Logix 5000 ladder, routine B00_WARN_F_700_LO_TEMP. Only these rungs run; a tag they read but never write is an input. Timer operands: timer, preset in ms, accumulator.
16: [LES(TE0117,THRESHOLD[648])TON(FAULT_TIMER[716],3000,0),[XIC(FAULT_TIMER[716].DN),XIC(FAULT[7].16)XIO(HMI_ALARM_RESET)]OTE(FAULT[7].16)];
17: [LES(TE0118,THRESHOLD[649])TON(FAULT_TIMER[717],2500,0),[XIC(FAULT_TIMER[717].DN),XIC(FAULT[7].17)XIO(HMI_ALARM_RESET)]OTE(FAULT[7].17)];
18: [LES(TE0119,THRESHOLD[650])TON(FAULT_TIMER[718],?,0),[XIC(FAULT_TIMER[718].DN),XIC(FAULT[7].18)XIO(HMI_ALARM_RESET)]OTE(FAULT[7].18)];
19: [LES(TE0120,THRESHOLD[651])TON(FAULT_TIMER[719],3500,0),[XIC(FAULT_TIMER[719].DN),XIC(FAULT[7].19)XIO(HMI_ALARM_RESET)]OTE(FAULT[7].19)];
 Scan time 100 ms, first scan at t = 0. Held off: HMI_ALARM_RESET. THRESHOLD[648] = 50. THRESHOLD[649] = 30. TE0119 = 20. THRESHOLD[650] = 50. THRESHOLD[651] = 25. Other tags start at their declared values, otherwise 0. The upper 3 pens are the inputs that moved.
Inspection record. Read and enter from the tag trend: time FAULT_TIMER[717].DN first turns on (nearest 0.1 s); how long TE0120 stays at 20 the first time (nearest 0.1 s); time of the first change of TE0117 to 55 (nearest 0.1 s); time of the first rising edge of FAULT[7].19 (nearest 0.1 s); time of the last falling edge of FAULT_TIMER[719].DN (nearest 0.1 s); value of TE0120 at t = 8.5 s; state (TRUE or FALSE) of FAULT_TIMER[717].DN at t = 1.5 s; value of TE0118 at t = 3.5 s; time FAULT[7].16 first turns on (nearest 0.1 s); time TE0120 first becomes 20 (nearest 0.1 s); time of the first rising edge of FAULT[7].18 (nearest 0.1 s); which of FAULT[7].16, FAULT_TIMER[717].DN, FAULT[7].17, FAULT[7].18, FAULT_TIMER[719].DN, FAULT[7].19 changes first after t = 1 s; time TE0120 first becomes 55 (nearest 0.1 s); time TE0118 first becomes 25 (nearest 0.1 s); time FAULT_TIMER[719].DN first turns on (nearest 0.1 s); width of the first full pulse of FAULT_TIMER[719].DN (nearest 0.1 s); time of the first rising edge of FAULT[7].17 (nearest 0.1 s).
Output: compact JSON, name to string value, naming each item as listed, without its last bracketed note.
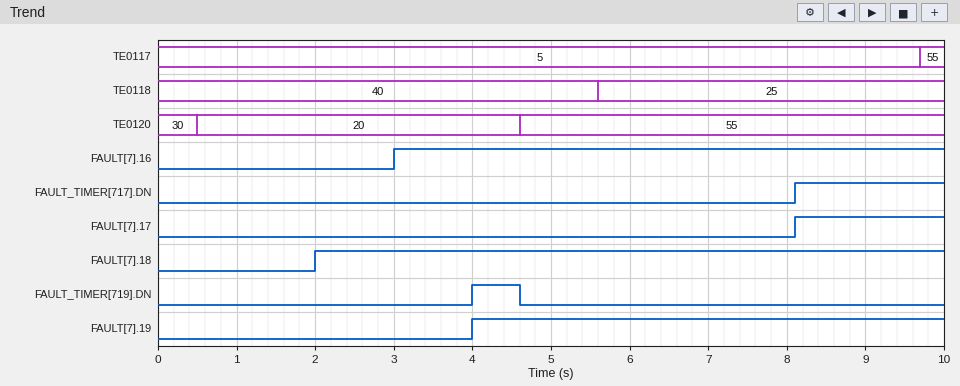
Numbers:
{"time FAULT_TIMER[717].DN first turns on": "8.1 s", "how long TE0120 stays at 20 the first time": "4.1 s", "time of the first change of TE0117 to 55": "9.7 s", "time of the first rising edge of FAULT[7].19": "4.0 s", "time of the last falling edge of FAULT_TIMER[719].DN": "4.6 s", "value of TE0120 at t = 8.5 s": "55", "state (TRUE or FALSE) of FAULT_TIMER[717].DN at t = 1.5 s": "FALSE", "value of TE0118 at t = 3.5 s": "40", "time FAULT[7].16 first turns on": "3.0 s", "time TE0120 first becomes 20": "0.5 s", "time of the first rising edge of FAULT[7].18": "2.0 s", "which of FAULT[7].16, FAULT_TIMER[717].DN, FAULT[7].17, FAULT[7].18, FAULT_TIMER[719].DN, FAULT[7].19 changes first after t = 1 s": "FAULT[7].18", "time TE0120 first becomes 55": "4.6 s", "time TE0118 first becomes 25": "5.6 s", "time FAULT_TIMER[719].DN first turns on": "4.0 s", "width of the first full pulse of FAULT_TIMER[719].DN": "0.6 s", "time of the first rising edge of FAULT[7].17": "8.1 s"}
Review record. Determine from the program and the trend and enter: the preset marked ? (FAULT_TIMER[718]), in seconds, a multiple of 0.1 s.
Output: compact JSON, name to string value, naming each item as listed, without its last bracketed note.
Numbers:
{"the preset marked ? (FAULT_TIMER[718]), in seconds, a multiple of 0.1 s": "2.0 s"}
